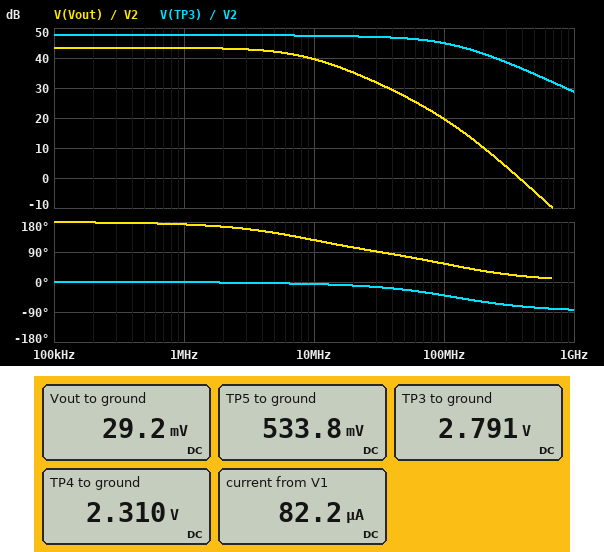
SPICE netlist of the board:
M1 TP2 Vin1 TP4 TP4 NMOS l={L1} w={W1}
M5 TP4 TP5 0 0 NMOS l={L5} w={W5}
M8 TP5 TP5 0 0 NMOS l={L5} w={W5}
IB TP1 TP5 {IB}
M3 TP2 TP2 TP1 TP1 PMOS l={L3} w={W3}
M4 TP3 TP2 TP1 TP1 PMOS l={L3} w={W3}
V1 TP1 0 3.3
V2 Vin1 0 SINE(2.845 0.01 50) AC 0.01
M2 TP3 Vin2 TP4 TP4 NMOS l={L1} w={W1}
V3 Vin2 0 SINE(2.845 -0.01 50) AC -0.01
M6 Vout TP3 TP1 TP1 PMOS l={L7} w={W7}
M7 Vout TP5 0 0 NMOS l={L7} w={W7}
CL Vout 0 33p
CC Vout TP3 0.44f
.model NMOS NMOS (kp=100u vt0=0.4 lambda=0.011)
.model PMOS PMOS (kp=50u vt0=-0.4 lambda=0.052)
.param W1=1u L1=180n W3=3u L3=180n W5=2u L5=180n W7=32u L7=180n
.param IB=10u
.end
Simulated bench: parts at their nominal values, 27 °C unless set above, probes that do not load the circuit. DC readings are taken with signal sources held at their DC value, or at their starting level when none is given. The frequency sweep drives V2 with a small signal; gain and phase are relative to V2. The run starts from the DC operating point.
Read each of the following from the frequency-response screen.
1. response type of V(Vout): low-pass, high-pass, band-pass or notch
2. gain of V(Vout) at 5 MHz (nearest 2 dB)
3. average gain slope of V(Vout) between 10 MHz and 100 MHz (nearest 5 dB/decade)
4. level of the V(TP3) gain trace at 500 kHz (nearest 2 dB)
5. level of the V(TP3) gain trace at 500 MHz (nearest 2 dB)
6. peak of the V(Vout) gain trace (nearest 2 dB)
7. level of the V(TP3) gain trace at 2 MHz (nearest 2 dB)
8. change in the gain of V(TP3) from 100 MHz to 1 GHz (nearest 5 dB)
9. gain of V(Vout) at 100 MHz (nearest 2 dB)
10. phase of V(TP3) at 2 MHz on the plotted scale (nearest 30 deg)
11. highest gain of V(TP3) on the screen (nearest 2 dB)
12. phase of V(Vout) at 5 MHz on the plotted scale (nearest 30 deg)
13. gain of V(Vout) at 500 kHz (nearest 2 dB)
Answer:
low-pass
42 dB
-20 dB/decade
48 dB
34 dB
44 dB
48 dB
-15 dB
20 dB
0 deg
48 dB
150 deg
44 dB
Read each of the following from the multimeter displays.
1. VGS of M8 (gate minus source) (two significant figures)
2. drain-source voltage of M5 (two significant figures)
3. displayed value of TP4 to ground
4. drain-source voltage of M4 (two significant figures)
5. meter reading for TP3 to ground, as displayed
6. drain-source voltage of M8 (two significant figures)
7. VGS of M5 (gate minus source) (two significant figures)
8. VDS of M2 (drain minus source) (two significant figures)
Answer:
530 mV
2.3 V
2.310 V
-510 mV
2.791 V
530 mV
530 mV
480 mV
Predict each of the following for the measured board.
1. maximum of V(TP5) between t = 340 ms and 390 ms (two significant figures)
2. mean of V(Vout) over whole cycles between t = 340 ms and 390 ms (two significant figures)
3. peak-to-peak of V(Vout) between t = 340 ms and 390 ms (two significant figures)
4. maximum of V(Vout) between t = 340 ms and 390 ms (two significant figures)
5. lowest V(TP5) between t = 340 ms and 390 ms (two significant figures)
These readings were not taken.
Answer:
530 mV
1.6 V
3.3 V
3.3 V
530 mV
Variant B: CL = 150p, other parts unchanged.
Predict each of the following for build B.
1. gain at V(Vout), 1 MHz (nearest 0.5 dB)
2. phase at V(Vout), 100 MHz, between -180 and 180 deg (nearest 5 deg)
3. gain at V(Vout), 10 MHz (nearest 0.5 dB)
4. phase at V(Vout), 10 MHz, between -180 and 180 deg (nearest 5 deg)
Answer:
42.5 dB
50 deg
29.0 dB
95 deg
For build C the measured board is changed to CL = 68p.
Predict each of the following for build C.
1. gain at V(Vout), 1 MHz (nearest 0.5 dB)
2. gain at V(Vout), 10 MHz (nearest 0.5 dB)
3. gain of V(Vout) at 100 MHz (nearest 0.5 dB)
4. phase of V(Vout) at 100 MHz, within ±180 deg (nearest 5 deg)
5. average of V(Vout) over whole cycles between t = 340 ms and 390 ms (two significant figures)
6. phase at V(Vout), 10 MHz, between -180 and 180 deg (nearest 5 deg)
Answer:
43.0 dB
35.0 dB
13.5 dB
50 deg
1.6 V
110 deg
